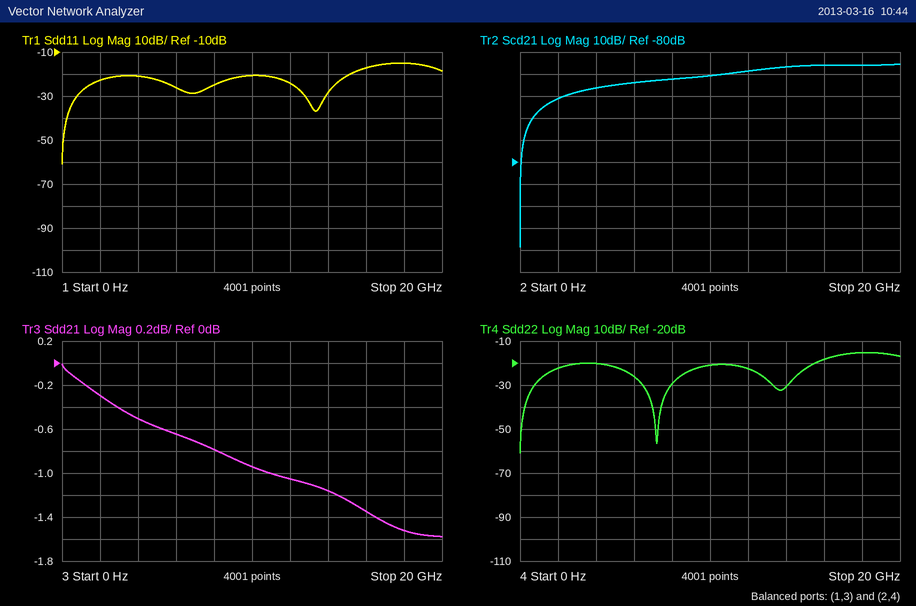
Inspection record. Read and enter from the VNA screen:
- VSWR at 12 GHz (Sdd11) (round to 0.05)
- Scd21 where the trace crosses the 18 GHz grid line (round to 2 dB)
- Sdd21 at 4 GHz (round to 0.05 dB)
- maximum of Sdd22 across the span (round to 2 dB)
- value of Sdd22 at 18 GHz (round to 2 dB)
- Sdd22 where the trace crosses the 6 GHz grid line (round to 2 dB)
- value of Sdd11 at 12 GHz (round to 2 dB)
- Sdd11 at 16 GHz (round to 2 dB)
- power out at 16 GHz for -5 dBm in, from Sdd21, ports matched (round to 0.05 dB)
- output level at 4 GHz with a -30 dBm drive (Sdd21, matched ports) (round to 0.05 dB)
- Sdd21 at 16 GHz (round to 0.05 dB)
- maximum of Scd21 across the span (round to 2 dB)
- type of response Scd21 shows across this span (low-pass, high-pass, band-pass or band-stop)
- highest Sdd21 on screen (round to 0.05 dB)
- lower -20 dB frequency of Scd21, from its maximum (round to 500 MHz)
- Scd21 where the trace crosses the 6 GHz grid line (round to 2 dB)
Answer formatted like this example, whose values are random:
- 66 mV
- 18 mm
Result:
- 1.15
- -36 dB
- -0.50 dB
- -16 dB
- -16 dB
- -26 dB
- -24 dB
- -18 dB
- -6.35 dBm
- -30.50 dBm
- -1.35 dB
- -36 dB
- high-pass
- 0.00 dB
- 1.0 GHz
- -44 dB
